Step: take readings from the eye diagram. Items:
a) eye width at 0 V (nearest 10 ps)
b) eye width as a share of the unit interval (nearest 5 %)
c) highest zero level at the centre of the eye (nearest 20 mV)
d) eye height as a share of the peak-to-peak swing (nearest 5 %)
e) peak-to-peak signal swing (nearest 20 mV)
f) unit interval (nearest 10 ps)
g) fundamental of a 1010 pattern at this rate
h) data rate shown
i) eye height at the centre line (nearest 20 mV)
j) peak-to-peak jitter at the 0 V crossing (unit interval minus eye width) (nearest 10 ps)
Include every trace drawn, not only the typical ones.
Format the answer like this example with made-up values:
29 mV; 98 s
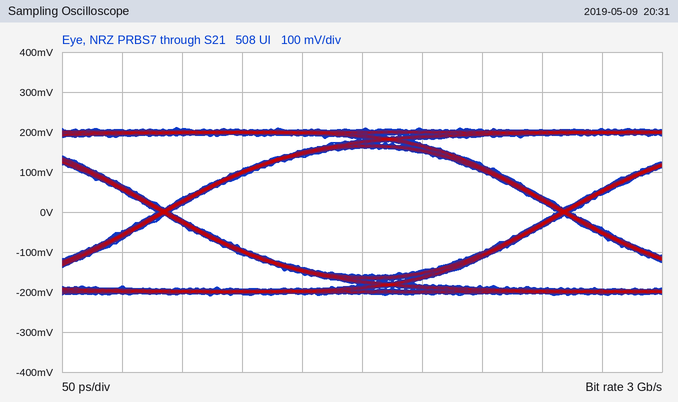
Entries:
320 ps; 95 %; -160 mV; 75 %; 420 mV; 330 ps; 1.5 GHz; 3 Gb/s; 320 mV; 10 ps
